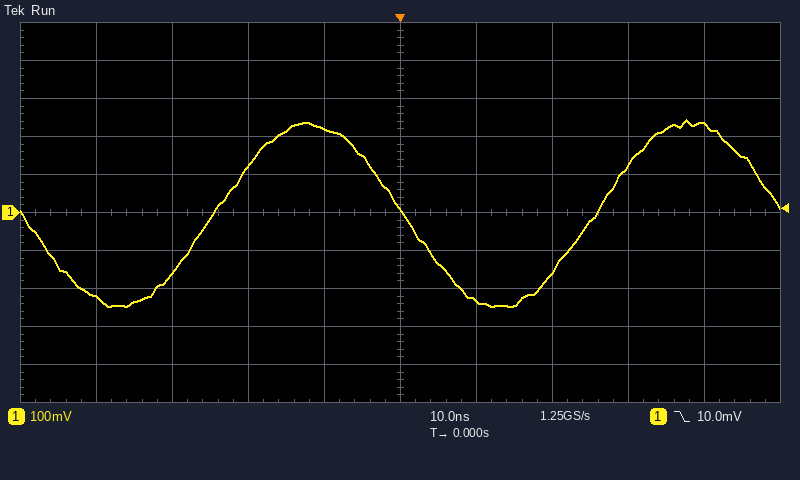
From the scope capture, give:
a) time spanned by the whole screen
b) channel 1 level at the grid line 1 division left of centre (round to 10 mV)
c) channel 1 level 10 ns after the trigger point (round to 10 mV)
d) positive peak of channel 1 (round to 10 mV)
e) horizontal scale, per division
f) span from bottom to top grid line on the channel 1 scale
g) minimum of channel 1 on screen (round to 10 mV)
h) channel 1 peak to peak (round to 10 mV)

100 ns
220 mV
-230 mV
240 mV
10 ns
1 V
-250 mV
490 mV
